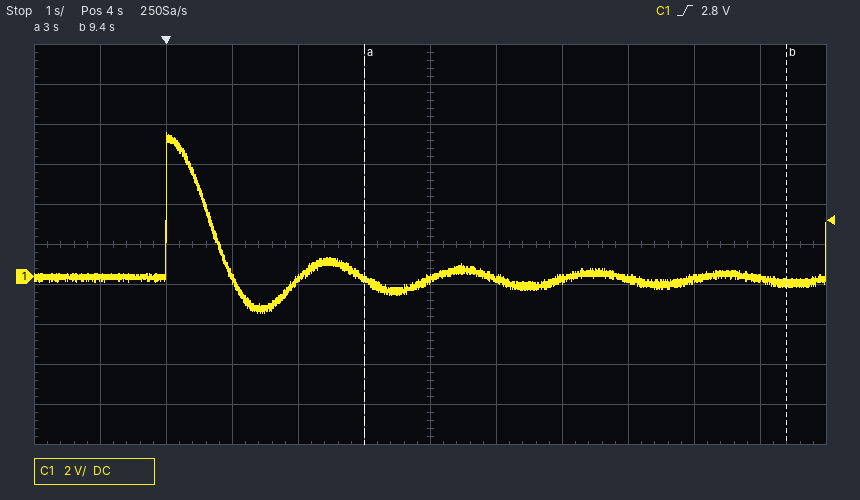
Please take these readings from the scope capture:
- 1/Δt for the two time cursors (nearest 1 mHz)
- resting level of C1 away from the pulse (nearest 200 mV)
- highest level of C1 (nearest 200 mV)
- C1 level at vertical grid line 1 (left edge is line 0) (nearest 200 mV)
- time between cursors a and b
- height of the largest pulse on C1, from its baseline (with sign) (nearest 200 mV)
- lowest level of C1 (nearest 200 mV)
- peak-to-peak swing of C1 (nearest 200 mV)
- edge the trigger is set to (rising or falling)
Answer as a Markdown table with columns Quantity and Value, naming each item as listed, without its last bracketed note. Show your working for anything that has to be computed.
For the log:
| Quantity | Value |
|---|---|
| 1/Δt for the two time cursors | 1 / 6.4 s ≈ 156 mHz |
| resting level of C1 away from the pulse | 0.0 V |
| highest level of C1 | 7.2 V |
| C1 level at vertical grid line 1 (left edge is line 0) | 0.0 V |
| time between cursors a and b | 9.4 s − (3 s) = 6.4 s |
| height of the largest pulse on C1, from its baseline (with sign) | 7.2 V − (0.0 V) = +7.2 V |
| lowest level of C1 | -1.8 V |
| peak-to-peak swing of C1 | 7.2 V − (-1.8 V) = 9.0 V |
| edge the trigger is set to | rising |
